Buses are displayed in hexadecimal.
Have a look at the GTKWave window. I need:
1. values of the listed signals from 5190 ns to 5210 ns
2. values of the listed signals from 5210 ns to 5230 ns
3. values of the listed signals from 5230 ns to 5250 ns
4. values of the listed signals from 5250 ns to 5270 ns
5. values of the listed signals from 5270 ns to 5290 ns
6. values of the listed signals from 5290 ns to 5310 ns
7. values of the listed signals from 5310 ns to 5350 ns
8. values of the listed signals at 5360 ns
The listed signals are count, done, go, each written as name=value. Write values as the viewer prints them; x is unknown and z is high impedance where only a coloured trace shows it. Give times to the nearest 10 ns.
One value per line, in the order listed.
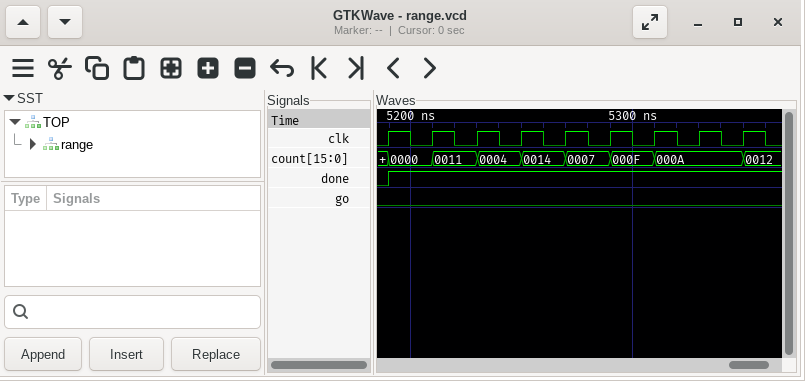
count=0000, done=1, go=0
count=0011, done=1, go=0
count=0004, done=1, go=0
count=0014, done=1, go=0
count=0007, done=1, go=0
count=000F, done=1, go=0
count=000A, done=1, go=0
count=0012, done=1, go=0
